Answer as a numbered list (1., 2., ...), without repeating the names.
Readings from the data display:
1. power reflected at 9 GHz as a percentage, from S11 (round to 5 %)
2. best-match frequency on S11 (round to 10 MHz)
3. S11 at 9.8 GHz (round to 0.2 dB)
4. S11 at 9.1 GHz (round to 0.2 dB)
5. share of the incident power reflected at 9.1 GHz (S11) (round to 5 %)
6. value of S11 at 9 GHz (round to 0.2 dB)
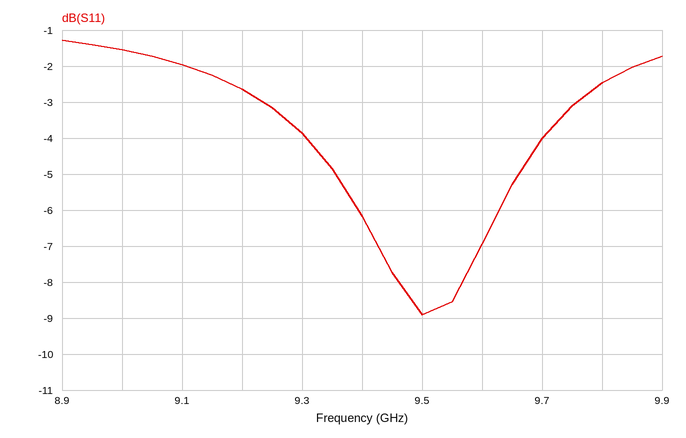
1. 70 %
2. 9.50 GHz
3. -2.4 dB
4. -2.0 dB
5. 65 %
6. -1.6 dB
